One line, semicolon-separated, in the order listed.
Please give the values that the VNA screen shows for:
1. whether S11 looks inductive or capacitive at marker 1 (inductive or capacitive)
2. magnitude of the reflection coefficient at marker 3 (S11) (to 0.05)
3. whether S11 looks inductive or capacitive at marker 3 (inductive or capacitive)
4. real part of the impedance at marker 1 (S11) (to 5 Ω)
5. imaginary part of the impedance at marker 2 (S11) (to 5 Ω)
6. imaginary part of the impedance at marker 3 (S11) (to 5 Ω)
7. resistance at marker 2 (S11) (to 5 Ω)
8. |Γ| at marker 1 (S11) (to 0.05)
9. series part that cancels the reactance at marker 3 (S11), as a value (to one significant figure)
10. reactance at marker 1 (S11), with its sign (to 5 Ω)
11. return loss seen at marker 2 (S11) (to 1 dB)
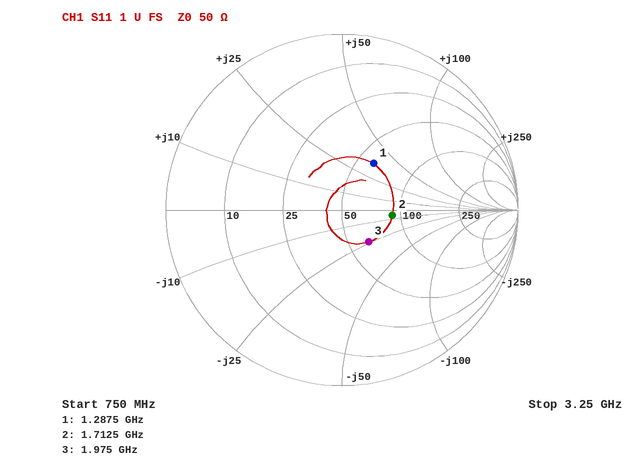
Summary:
inductive; 0.25; capacitive; 60 Ω; -5 Ω; -25 Ω; 90 Ω; 0.30; 2 nH; +35 Ω; 11 dB
